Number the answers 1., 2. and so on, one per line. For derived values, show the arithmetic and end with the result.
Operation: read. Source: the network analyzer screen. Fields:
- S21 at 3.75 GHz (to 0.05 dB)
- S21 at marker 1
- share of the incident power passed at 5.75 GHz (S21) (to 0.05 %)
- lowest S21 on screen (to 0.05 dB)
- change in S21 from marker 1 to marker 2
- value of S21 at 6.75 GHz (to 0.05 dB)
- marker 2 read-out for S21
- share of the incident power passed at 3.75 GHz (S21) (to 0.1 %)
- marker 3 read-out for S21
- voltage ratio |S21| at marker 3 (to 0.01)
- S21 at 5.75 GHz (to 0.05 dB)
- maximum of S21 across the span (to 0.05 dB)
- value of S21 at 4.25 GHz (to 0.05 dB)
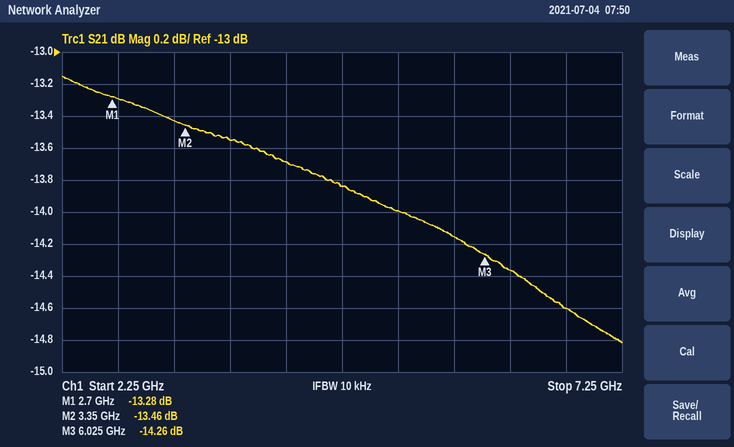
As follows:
1. -13.55 dB
2. -13.28 dB
3. 10^(-14.15/10) ≈ 3.85 %
4. -14.80 dB
5. -13.46 − (-13.28) = -0.18 dB
6. -14.60 dB
7. -13.46 dB
8. 10^(-13.55/10) ≈ 4.4 %
9. -14.26 dB
10. 10^(-14.26/20) ≈ 0.19
11. -14.15 dB
12. -13.15 dB
13. -13.70 dB
